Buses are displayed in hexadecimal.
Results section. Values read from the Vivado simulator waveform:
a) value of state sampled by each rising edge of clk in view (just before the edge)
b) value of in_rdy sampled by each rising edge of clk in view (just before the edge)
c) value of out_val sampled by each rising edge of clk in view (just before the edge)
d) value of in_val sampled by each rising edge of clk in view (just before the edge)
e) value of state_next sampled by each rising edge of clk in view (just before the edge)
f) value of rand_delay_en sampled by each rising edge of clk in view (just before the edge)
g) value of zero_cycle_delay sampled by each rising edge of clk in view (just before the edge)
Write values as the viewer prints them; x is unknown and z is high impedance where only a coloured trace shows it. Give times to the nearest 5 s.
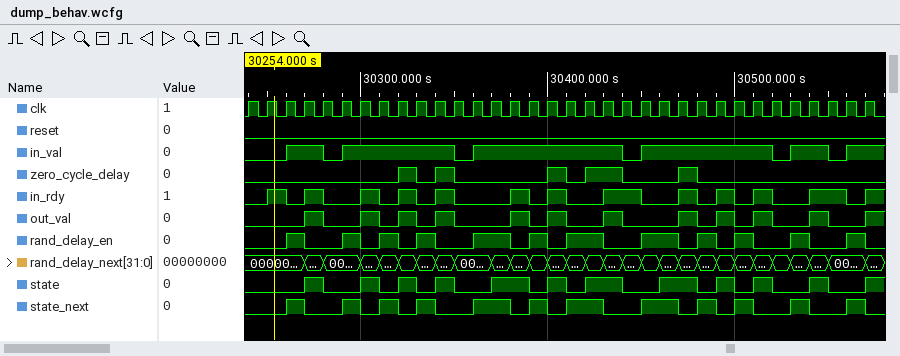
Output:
0 0 0 0 1 0 0 1 0 1 0 1 0 0 1 1 0 1 0 1 1 0 0 1 1 0 1 0 1 0 0 1 0 0
0 0 1 0 1 0 0 1 0 1 0 1 0 0 0 1 0 1 0 0 1 1 0 0 1 0 1 0 1 0 0 1 1 0
0 0 0 0 1 0 0 1 0 1 0 1 0 0 0 1 0 1 0 0 1 0 0 0 1 0 1 0 1 0 0 1 0 0
0 0 0 1 1 0 1 1 1 1 1 1 0 1 1 1 1 1 1 1 1 0 1 1 1 1 1 1 1 0 1 1 0 1
0 0 0 1 0 0 1 0 1 0 1 0 0 1 1 0 1 0 1 1 0 0 1 1 0 1 0 1 0 0 1 0 0 1
0 0 0 1 0 0 1 0 1 0 1 0 0 1 1 0 1 0 1 1 0 0 1 1 0 1 0 1 0 0 1 0 0 1
0 0 0 0 0 0 0 0 0 1 0 1 0 0 0 0 0 1 0 1 1 0 0 0 1 0 0 0 0 0 0 0 0 0
